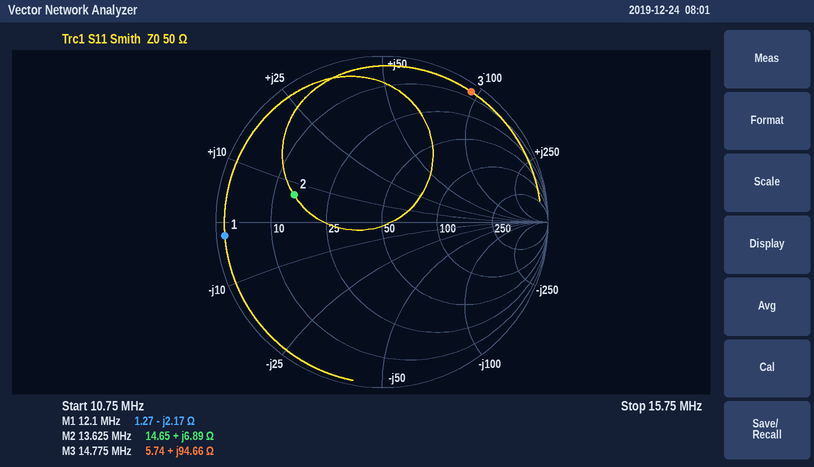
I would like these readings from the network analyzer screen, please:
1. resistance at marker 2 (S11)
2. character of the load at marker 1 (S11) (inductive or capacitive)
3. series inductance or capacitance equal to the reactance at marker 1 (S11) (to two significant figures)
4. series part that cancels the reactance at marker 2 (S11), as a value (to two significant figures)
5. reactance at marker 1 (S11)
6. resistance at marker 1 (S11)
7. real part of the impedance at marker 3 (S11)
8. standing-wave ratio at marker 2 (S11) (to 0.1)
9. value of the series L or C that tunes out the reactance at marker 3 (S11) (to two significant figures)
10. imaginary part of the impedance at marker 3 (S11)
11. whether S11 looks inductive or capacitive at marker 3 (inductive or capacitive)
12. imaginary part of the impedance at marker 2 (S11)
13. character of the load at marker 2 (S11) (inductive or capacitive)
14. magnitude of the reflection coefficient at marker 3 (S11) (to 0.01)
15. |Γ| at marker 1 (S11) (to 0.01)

14.65 Ω
capacitive
6.1 nF
1.7 nF
-2.17 Ω
1.27 Ω
5.74 Ω
3.5
110 pF
+94.66 Ω
inductive
+6.89 Ω
inductive
0.95
0.95
